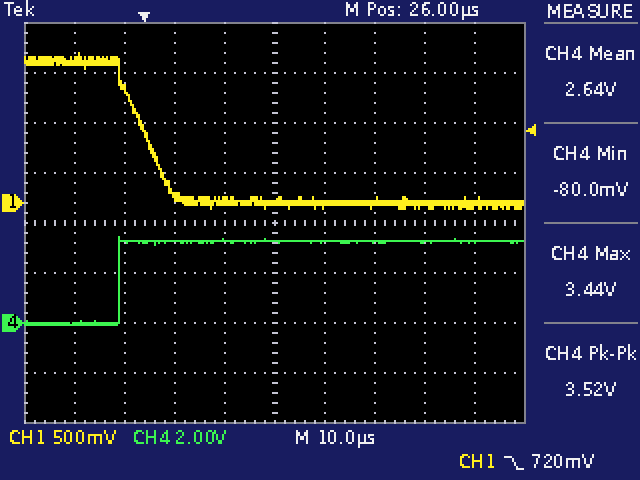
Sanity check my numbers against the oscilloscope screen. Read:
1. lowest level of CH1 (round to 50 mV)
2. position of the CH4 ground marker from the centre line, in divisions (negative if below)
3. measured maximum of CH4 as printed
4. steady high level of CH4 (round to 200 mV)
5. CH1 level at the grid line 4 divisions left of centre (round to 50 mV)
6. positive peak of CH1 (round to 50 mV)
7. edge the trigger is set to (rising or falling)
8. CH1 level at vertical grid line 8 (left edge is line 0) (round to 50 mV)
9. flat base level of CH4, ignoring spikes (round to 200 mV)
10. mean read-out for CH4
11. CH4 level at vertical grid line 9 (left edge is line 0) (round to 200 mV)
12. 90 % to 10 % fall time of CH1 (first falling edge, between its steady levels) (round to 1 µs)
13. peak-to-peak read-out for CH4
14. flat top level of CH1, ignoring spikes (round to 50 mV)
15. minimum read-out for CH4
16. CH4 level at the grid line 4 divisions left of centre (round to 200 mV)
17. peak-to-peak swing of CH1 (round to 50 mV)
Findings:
-50 mV
-2.0 div
3.44 V
3.2 V
1.40 V
1.50 V
falling
0 mV
0.0 V
2.64 V
3.2 V
10 µs
3.52 V
1.40 V
-80.0 mV
0.0 V
1.55 V
